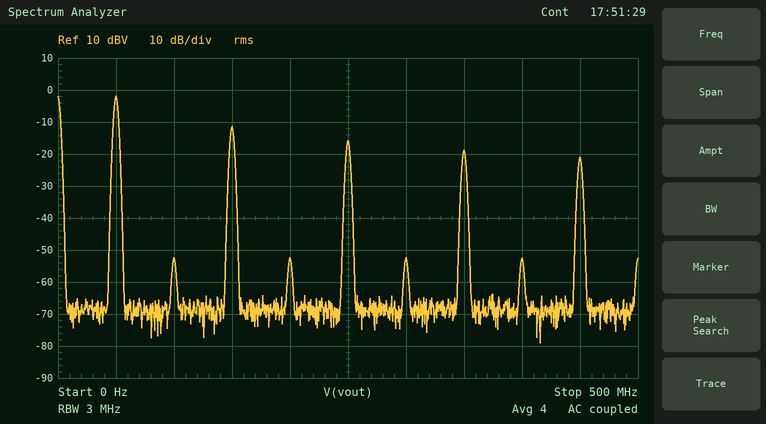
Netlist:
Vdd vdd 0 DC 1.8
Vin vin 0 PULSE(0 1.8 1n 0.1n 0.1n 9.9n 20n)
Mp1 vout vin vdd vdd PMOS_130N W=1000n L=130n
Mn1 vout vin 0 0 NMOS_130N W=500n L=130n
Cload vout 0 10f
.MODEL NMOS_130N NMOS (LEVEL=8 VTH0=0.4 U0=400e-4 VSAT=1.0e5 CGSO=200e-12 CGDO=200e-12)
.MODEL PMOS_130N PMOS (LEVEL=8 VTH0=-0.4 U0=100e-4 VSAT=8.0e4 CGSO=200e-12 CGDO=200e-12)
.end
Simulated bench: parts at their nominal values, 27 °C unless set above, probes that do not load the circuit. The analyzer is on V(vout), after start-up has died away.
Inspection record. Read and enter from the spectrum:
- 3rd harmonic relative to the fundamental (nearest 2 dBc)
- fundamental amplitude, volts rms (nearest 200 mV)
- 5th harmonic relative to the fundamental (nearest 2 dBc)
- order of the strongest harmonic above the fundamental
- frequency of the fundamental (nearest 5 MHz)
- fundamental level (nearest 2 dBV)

-10 dBc
800 mV
-14 dBc
3
50 MHz
-2 dBV
